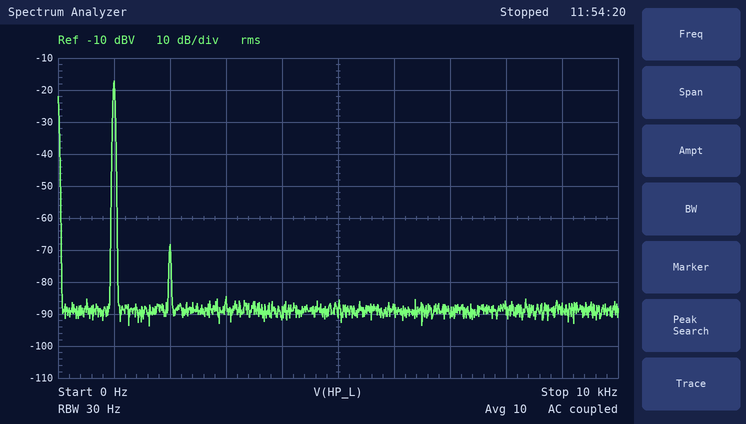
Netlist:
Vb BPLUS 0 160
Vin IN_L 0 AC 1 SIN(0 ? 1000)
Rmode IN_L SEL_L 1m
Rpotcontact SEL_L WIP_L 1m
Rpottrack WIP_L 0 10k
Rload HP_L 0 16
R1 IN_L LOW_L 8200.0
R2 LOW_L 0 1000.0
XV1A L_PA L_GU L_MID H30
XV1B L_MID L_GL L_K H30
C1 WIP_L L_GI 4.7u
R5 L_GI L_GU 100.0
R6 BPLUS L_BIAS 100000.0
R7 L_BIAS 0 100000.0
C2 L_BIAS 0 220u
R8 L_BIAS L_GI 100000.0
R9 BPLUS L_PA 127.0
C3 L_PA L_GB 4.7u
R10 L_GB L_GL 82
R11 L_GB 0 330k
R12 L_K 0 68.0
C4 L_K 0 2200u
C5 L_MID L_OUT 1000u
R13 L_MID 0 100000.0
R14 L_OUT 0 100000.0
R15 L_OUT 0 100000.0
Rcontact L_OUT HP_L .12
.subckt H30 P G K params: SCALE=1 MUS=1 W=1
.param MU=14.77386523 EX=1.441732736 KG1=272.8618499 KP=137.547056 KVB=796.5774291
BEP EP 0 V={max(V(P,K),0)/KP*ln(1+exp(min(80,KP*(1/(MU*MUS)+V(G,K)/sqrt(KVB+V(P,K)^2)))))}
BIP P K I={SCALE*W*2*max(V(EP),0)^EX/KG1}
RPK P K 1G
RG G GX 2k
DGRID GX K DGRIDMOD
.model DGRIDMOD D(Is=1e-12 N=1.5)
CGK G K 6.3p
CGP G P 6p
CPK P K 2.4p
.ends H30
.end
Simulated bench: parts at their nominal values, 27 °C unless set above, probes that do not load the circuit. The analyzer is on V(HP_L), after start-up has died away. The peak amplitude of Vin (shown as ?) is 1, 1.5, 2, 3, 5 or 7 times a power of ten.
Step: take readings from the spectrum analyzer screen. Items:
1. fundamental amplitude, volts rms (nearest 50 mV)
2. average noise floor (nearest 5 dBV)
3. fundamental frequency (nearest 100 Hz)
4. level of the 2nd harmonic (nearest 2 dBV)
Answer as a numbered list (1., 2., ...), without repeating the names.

1. 150 mV
2. -90 dBV
3. 1.0 kHz
4. -68 dBV
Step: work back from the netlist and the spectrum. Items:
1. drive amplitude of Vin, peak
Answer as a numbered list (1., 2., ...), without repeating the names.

1. 500 mV
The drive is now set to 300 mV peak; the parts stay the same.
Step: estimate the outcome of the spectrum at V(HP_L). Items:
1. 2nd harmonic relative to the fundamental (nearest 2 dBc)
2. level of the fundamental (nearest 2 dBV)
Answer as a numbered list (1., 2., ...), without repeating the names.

1. -56 dBc
2. -22 dBV
